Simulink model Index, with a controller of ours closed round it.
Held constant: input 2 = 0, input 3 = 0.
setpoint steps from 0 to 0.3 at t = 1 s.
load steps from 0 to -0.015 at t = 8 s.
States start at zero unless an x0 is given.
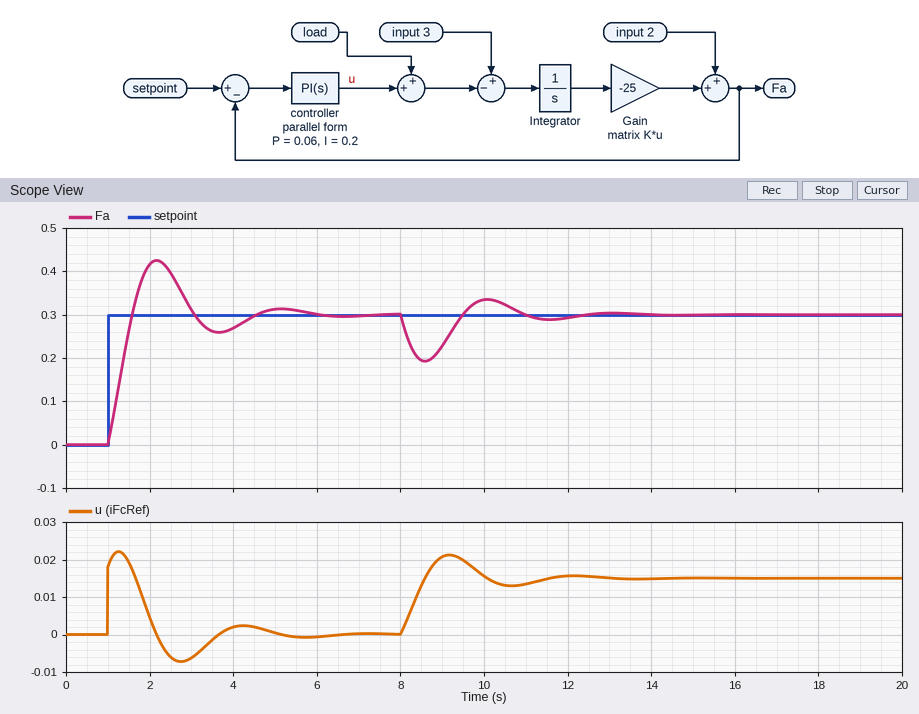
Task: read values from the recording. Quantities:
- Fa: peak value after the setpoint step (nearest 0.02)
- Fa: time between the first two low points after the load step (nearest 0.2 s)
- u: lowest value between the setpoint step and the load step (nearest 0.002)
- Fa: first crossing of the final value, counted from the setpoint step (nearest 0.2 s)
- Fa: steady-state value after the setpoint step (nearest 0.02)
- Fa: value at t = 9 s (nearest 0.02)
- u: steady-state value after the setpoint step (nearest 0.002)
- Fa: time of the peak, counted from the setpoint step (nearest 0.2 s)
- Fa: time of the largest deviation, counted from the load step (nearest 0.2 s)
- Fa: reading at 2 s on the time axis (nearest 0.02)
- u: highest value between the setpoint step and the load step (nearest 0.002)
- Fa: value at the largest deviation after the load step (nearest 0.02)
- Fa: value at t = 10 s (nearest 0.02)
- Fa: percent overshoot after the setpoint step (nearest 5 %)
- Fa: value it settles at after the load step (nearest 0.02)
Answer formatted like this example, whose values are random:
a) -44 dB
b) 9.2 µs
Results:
a) 0.42
b) 3.0 s
c) -0.008
d) 0.6 s
e) 0.30
f) 0.22
g) 0.000
h) 1.2 s
i) 0.6 s
j) 0.42
k) 0.022
l) 0.20
m) 0.34
n) 40 %
o) 0.30
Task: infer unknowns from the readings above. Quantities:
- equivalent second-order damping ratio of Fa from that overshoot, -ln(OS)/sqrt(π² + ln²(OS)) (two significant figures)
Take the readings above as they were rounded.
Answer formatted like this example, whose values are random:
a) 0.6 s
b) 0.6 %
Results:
a) 0.28
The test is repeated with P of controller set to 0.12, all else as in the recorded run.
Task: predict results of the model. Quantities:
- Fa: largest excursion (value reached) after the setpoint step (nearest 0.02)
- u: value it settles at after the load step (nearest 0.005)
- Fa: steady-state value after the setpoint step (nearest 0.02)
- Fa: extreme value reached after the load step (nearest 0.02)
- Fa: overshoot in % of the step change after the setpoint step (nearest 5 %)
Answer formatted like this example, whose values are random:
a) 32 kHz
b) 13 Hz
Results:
a) 0.36
b) 0.015
c) 0.30
d) 0.22
e) 20 %
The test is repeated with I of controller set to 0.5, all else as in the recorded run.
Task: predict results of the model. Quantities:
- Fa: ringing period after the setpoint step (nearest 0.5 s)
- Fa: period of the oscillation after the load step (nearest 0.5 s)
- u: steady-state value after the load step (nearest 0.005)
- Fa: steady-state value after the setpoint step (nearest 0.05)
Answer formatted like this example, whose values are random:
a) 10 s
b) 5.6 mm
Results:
a) 2.0 s
b) 2.0 s
c) 0.015
d) 0.30
